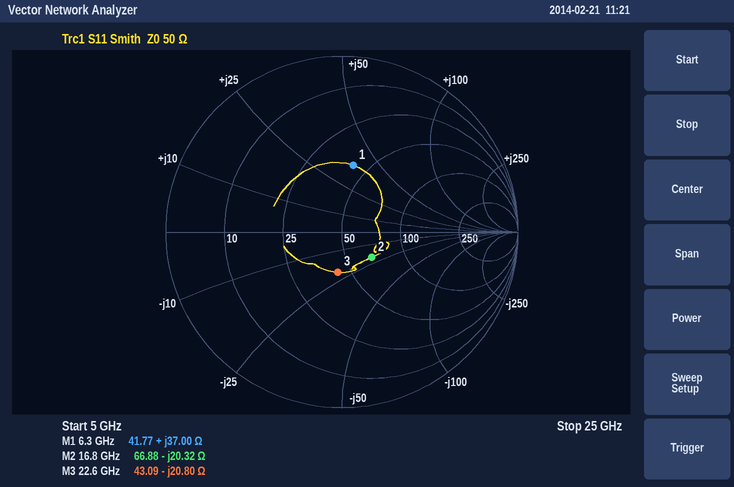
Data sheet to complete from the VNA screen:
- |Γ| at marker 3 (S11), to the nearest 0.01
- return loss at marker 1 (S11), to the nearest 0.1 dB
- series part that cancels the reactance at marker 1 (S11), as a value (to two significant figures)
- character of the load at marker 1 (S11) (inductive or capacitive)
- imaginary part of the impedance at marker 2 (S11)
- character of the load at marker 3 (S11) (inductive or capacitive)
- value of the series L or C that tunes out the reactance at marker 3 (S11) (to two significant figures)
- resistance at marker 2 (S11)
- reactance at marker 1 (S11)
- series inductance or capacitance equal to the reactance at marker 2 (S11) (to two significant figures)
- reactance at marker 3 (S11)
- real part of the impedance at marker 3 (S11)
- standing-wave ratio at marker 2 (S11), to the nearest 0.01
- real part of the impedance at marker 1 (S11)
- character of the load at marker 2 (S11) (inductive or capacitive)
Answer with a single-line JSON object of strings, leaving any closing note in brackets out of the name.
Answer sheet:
{"|Γ| at marker 3 (S11), to the nearest 0.01": "0.23", "return loss at marker 1 (S11), to the nearest 0.1 dB": "8.3 dB", "series part that cancels the reactance at marker 1 (S11), as a value": "680 fF", "character of the load at marker 1 (S11)": "inductive", "imaginary part of the impedance at marker 2": "-20.32 Ω", "character of the load at marker 3 (S11)": "capacitive", "value of the series L or C that tunes out the reactance at marker 3 (S11)": "150 pH", "resistance at marker 2": "66.88 Ω", "reactance at marker 1": "+37.00 Ω", "series inductance or capacitance equal to the reactance at marker 2 (S11)": "470 fF", "reactance at marker 3": "-20.80 Ω", "real part of the impedance at marker 3": "43.09 Ω", "standing-wave ratio at marker 2 (S11), to the nearest 0.01": "1.57", "real part of the impedance at marker 1": "41.77 Ω", "character of the load at marker 2 (S11)": "capacitive"}
